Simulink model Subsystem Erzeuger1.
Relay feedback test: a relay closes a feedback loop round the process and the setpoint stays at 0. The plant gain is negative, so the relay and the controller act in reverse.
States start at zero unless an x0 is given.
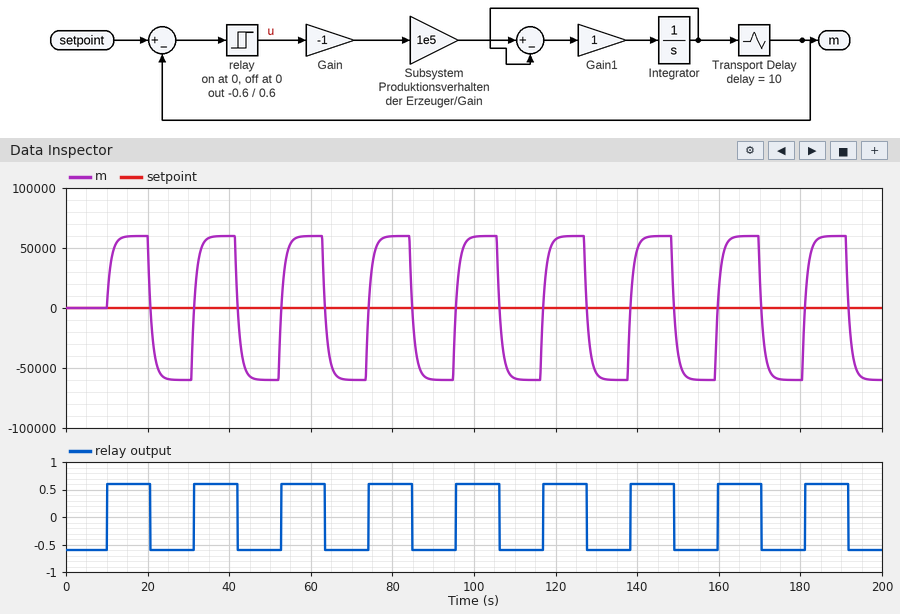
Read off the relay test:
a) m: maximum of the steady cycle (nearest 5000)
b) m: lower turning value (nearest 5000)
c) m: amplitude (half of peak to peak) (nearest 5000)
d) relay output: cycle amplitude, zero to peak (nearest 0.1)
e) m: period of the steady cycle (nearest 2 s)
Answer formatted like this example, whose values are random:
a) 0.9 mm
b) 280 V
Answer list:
a) 60000
b) -60000
c) 60000
d) 0.6
e) 22 s
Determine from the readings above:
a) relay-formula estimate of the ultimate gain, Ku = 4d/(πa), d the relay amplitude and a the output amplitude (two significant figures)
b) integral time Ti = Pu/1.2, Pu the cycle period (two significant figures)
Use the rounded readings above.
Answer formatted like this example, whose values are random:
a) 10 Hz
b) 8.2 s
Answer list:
a) 0.000013
b) 18 s
